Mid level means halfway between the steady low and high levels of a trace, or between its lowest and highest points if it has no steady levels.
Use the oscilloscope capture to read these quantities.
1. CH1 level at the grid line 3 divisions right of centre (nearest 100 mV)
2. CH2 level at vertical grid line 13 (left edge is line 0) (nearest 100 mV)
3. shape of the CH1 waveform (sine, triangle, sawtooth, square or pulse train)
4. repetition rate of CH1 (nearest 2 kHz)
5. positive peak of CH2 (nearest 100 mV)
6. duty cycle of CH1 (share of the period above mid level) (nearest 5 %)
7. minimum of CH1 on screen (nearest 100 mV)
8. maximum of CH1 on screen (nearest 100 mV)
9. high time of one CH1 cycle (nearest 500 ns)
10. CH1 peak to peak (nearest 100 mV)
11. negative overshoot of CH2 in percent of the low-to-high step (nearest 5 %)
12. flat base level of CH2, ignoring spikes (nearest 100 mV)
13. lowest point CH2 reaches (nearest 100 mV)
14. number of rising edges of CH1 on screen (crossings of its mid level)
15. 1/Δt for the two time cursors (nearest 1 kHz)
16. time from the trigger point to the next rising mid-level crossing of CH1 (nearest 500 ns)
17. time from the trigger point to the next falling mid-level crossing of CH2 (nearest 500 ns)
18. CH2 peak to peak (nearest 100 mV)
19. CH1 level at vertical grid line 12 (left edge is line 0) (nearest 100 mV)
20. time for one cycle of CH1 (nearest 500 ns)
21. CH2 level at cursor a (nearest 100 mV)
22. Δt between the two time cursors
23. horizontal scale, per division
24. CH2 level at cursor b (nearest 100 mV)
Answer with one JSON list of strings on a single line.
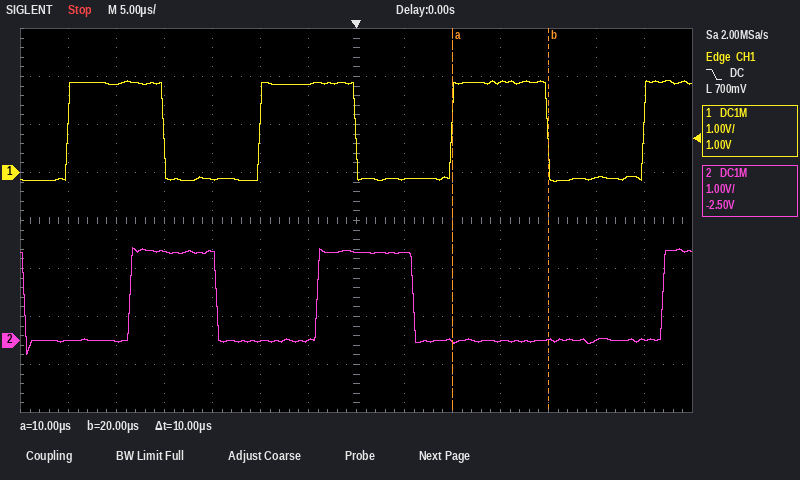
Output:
["1.9 V", "0.0 V", "square", "50 kHz", "1.9 V", "50 %", "-200 mV", "1.9 V", "10.0 µs", "2.1 V", "15 %", "0.0 V", "-300 mV", "4", "100 kHz", "10.0 µs", "6.0 µs", "2.2 V", "-100 mV", "20.0 µs", "0.0 V", "10 µs", "5 µs", "0.0 V"]
